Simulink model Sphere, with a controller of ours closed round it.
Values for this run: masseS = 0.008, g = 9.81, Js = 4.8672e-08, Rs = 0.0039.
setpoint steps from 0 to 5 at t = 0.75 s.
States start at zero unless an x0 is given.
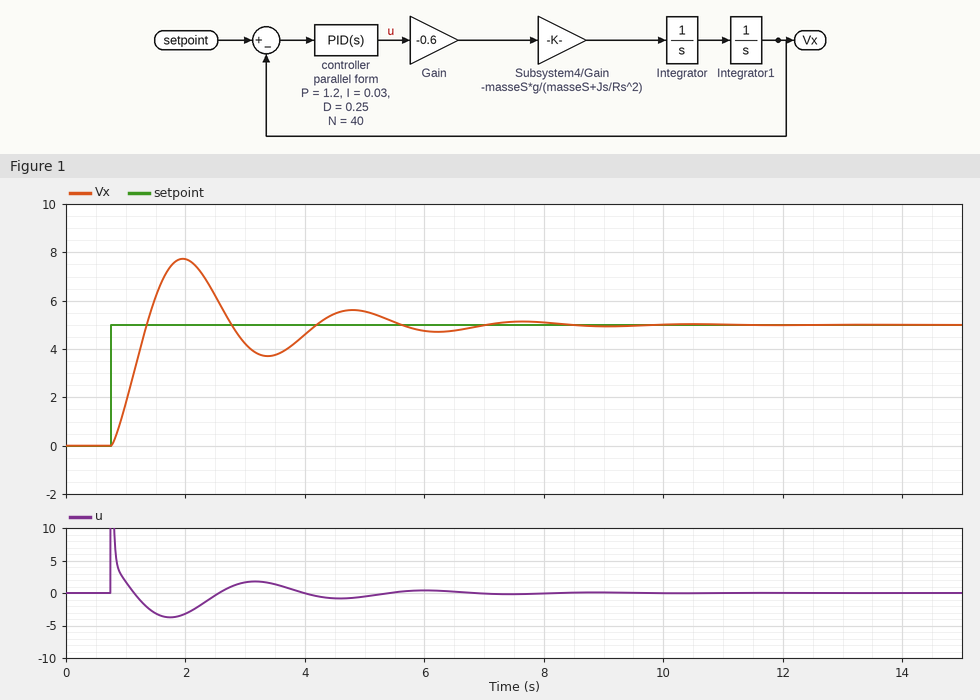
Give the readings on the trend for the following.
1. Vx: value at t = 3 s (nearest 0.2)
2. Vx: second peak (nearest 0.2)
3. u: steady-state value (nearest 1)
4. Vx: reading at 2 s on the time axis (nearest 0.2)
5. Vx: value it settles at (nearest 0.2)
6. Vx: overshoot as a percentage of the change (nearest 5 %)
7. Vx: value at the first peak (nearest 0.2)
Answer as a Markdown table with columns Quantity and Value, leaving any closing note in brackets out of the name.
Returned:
| Quantity | Value |
|---|---|
| Vx: value at t = 3 s | 4.2 |
| Vx: second peak | 5.6 |
| u: steady-state value | 0 |
| Vx: reading at 2 s on the time axis | 7.8 |
| Vx: value it settles at | 5.0 |
| Vx: overshoot as a percentage of the change | 55 % |
| Vx: value at the first peak | 7.8 |
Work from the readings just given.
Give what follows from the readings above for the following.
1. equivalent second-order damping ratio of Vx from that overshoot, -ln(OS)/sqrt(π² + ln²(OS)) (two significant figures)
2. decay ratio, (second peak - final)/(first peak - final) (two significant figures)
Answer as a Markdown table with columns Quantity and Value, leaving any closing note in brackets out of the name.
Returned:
| Quantity | Value |
|---|---|
| equivalent second-order damping ratio of Vx from that overshoot, -ln(OS)/sqrt(π² + ln²(OS)) | 0.19 |
| decay ratio, (second peak - final)/(first peak - final) | 0.21 |
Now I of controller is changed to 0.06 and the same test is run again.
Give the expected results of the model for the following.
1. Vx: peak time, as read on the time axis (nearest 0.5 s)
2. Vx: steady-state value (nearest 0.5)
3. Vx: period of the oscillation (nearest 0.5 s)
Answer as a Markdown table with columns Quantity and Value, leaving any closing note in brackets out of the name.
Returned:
| Quantity | Value |
|---|---|
| Vx: peak time, as read on the time axis | 2.0 s |
| Vx: steady-state value | 5.0 |
| Vx: period of the oscillation | 3.0 s |
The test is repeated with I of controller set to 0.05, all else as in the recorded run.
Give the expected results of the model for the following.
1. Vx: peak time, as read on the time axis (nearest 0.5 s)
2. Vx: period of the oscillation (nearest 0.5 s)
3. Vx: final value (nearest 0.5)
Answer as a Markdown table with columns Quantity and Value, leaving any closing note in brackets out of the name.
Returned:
| Quantity | Value |
|---|---|
| Vx: peak time, as read on the time axis | 2.0 s |
| Vx: period of the oscillation | 3.0 s |
| Vx: final value | 5.0 |
